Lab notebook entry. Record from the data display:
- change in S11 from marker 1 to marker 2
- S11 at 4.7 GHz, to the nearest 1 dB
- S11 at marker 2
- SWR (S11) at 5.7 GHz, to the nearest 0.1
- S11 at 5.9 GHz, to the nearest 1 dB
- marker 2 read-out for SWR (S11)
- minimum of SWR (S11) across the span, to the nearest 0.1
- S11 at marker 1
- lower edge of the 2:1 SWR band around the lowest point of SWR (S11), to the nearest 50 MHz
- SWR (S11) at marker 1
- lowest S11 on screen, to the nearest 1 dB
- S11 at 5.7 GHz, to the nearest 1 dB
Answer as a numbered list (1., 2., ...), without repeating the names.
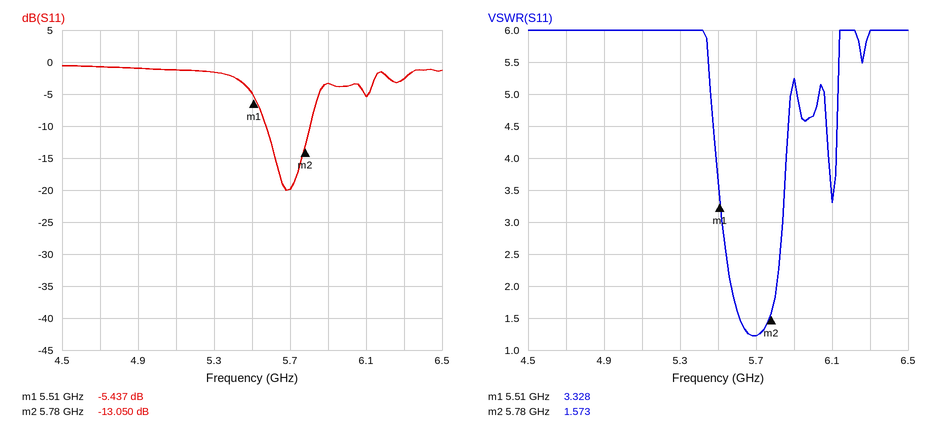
1. -7.613 dB
2. -1 dB
3. -13.050 dB
4. 1.2
5. -3 dB
6. 1.573
7. 1.2
8. -5.437 dB
9. 5.55 GHz
10. 3.328
11. -20 dB
12. -20 dB
